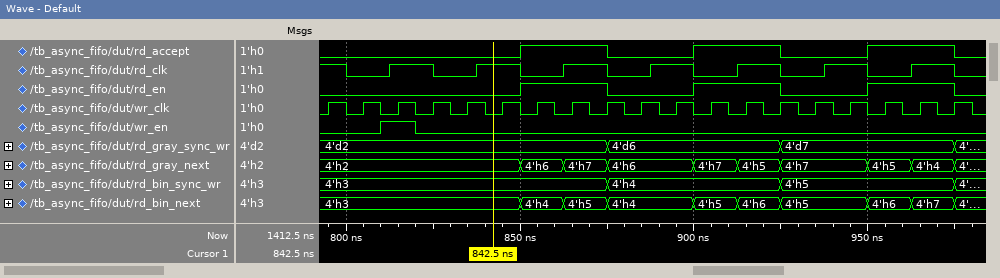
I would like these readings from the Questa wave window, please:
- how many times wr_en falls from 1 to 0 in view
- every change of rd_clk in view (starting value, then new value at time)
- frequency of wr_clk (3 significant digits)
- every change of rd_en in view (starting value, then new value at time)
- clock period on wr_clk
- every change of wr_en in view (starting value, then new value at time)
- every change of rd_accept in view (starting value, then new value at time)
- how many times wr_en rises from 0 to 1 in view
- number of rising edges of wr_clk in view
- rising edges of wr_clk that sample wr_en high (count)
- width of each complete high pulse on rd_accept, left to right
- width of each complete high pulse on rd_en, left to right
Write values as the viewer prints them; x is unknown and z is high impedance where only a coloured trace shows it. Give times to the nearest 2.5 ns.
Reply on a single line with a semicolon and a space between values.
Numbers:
1; 1, 0 at 800 ns, 1 at 812.5 ns, 0 at 825 ns, 1 at 837.5 ns, 0 at 850 ns, 1 at 862.5 ns, 0 at 875 ns, 1 at 887.5 ns, 0 at 900 ns, 1 at 912.5 ns, 0 at 925 ns, 1 at 937.5 ns, 0 at 950 ns, 1 at 962.5 ns, 0 at 975 ns; 100 MHz; 0, 1 at 850 ns, 0 at 875 ns, 1 at 900 ns, 0 at 925 ns, 1 at 950 ns, 0 at 975 ns; 10 ns; 0, 1 at 810 ns, 0 at 820 ns; 0, 1 at 850 ns, 0 at 875 ns, 1 at 900 ns, 0 at 925 ns, 1 at 950 ns, 0 at 975 ns; 1; 19; 1; 25 ns, 25 ns, 25 ns; 25 ns, 25 ns, 25 ns
